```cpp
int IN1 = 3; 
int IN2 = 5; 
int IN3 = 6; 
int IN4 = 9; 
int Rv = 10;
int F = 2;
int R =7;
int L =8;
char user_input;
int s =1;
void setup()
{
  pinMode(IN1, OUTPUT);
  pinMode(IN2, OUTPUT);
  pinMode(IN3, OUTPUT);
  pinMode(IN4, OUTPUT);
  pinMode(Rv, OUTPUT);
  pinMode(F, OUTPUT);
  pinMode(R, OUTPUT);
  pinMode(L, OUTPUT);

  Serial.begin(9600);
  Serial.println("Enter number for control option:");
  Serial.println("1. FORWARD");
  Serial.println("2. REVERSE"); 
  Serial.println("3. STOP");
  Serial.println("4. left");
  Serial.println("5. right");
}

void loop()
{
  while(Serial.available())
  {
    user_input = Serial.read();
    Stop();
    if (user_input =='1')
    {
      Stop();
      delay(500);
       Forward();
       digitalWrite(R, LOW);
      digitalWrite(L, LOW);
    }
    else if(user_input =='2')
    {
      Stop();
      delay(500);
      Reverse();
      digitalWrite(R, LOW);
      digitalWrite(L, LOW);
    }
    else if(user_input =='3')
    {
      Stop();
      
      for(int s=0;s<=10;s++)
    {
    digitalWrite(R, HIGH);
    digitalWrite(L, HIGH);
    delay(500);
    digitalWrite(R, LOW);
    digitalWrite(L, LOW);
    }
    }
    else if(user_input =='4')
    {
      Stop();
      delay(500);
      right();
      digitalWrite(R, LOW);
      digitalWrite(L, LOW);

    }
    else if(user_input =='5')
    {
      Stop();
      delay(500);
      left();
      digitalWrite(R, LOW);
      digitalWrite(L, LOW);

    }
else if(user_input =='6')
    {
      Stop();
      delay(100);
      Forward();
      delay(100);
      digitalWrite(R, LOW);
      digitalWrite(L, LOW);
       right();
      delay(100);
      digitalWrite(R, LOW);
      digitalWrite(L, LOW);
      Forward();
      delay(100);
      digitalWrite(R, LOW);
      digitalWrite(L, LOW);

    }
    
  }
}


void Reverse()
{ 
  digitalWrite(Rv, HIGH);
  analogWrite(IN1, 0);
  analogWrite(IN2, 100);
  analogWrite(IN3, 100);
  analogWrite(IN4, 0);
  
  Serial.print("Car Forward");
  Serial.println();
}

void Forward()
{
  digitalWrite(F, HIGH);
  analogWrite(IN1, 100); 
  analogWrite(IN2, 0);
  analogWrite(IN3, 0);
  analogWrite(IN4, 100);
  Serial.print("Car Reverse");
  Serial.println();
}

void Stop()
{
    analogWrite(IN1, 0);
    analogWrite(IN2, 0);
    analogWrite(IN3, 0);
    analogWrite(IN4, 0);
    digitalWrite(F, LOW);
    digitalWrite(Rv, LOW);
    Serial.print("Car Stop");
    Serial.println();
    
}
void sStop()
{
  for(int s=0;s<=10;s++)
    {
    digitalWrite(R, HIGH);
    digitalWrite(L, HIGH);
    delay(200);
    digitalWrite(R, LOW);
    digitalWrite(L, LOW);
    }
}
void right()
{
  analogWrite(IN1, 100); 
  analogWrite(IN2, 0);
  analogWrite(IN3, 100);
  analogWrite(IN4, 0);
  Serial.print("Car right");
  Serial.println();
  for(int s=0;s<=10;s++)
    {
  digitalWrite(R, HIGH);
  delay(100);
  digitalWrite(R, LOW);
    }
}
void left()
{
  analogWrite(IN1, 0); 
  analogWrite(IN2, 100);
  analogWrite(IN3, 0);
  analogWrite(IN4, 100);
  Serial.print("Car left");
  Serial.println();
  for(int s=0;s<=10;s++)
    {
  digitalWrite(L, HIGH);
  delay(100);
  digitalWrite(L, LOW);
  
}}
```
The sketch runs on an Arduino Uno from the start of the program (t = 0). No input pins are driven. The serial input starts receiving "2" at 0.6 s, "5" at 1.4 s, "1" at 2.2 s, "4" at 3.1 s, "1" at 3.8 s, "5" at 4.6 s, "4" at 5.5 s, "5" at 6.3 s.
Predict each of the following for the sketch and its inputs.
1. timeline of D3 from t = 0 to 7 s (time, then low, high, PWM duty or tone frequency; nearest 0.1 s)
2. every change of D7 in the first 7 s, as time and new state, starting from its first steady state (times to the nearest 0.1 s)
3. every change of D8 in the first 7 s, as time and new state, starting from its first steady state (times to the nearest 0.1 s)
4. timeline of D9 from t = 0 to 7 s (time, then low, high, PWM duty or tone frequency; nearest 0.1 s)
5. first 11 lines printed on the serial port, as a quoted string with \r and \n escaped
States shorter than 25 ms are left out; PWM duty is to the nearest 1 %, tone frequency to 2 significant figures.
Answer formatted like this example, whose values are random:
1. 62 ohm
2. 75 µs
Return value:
1. 0 s low; 4 s PWM 39 %; 5.1 s low
2. 0 s low; 4 s high; 5.1 s low
3. 0 s low; 1.9 s high; 3 s low; 6.1 s high
4. 0 s low; 1.9 s PWM 39 %; 3 s low; 6.1 s PWM 39 %
5. "Enter number for control option:\r\n1. FORWARD\r\n2. REVERSE\r\n3. STOP\r\n4. left\r\n5. right\r\nCar Stop\r\nCar Stop\r\nCar Forward\r\nCar Stop\r\nCar Stop\r\n"
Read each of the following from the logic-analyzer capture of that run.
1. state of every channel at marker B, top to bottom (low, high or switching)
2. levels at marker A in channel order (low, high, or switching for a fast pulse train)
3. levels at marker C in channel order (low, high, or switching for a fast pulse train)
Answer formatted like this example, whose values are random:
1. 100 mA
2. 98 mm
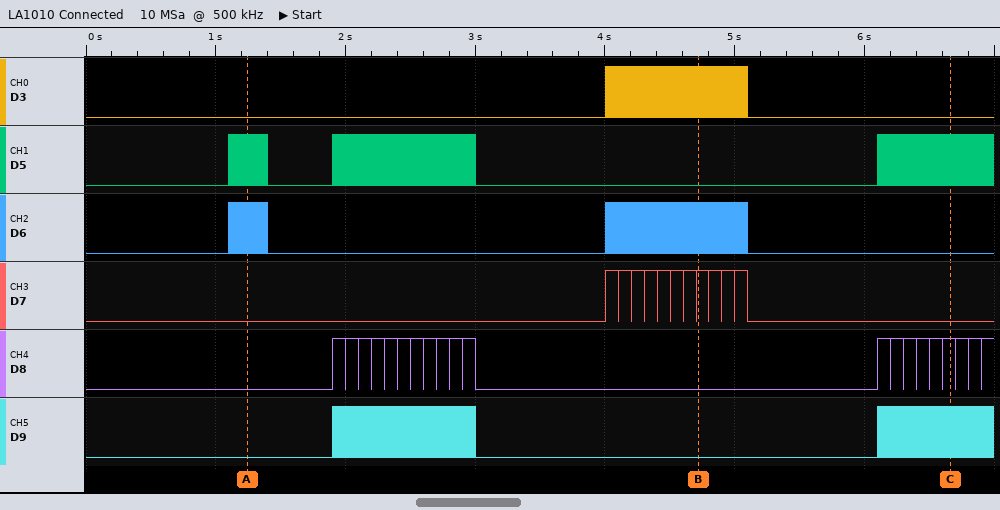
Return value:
1. D3 switching, D5 low, D6 switching, D7 high, D8 low, D9 low
2. D3 low, D5 switching, D6 switching, D7 low, D8 low, D9 low
3. D3 low, D5 switching, D6 low, D7 low, D8 high, D9 switching
